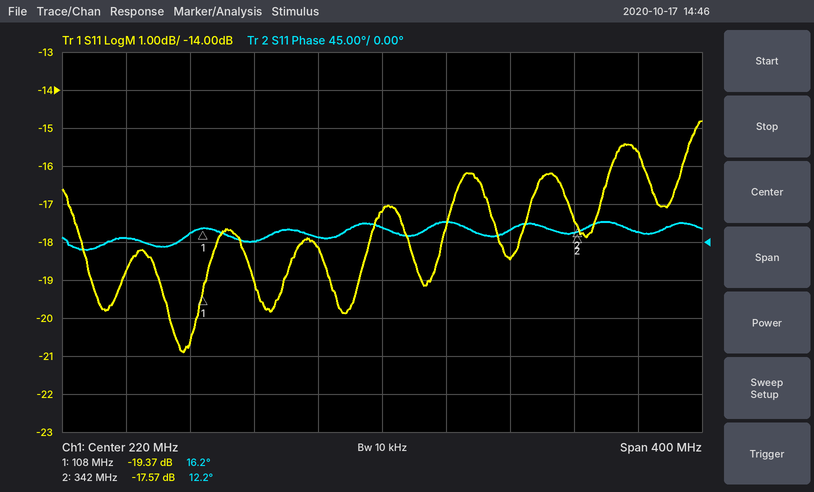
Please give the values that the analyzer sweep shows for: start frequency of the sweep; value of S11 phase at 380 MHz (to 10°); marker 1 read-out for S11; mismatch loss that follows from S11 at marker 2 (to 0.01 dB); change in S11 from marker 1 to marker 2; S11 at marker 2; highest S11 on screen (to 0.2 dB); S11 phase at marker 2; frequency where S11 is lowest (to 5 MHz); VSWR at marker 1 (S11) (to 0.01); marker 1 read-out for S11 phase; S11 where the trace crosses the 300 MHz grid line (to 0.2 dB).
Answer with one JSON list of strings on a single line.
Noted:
["20 MHz", "10°", "-19.37 dB", "0.08 dB", "1.80 dB", "-17.57 dB", "-14.8 dB", "12.2°", "95 MHz", "1.24", "16.2°", "-18.4 dB"]
